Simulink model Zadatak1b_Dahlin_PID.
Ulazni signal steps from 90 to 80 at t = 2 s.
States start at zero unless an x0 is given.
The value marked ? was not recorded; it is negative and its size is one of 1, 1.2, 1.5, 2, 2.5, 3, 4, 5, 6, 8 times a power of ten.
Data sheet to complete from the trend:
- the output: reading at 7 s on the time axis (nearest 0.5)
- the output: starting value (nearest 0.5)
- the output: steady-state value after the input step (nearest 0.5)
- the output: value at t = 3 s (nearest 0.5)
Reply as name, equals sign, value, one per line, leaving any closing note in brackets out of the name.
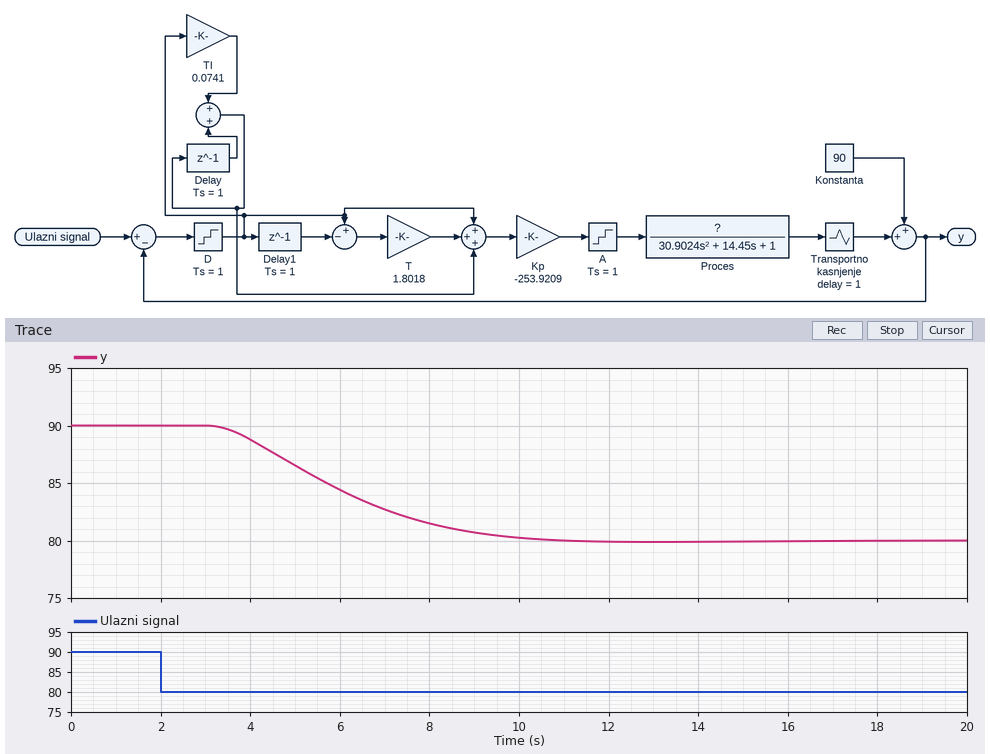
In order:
the output: reading at 7 s on the time axis = 82.5
the output: starting value = 90.0
the output: steady-state value after the input step = 80.0
the output: value at t = 3 s = 90.0
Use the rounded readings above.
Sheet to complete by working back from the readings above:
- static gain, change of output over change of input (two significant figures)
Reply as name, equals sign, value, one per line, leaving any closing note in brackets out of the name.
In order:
static gain, change of output over change of input = 1.0
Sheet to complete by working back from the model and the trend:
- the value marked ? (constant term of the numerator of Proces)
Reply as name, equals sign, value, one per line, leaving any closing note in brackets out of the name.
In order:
the value marked ? = -0.012
